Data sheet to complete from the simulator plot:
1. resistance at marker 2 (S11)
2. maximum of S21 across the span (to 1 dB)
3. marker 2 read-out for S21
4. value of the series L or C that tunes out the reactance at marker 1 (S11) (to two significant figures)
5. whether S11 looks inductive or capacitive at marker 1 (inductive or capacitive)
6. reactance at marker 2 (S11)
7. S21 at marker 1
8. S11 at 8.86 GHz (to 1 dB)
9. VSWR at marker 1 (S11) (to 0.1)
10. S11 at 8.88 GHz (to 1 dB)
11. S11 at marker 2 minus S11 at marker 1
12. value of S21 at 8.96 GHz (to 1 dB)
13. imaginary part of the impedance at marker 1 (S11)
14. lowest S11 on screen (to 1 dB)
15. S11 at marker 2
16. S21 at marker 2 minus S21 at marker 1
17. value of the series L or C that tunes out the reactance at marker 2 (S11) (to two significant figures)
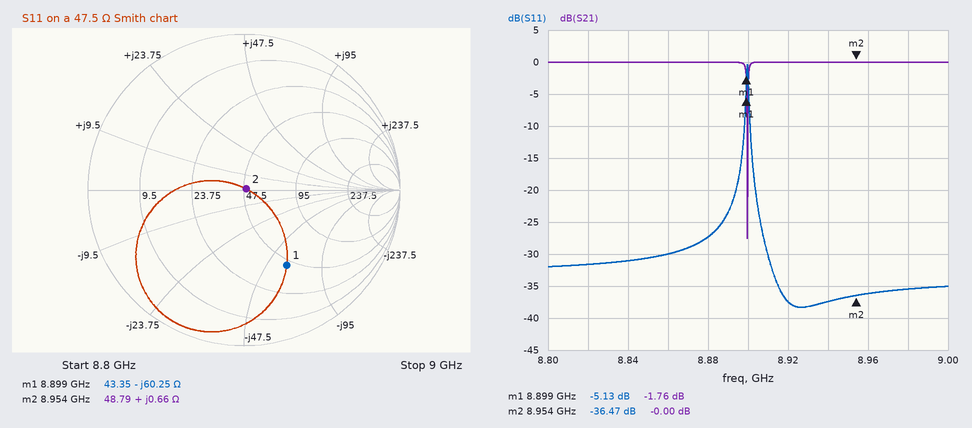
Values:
48.79 Ω
0 dB
-0.00 dB
1.1 nH
capacitive
+0.66 Ω
-1.76 dB
-30 dB
3.5
-27 dB
-31.34 dB
0 dB
-60.25 Ω
-38 dB
-36.47 dB
1.76 dB
27 pF
